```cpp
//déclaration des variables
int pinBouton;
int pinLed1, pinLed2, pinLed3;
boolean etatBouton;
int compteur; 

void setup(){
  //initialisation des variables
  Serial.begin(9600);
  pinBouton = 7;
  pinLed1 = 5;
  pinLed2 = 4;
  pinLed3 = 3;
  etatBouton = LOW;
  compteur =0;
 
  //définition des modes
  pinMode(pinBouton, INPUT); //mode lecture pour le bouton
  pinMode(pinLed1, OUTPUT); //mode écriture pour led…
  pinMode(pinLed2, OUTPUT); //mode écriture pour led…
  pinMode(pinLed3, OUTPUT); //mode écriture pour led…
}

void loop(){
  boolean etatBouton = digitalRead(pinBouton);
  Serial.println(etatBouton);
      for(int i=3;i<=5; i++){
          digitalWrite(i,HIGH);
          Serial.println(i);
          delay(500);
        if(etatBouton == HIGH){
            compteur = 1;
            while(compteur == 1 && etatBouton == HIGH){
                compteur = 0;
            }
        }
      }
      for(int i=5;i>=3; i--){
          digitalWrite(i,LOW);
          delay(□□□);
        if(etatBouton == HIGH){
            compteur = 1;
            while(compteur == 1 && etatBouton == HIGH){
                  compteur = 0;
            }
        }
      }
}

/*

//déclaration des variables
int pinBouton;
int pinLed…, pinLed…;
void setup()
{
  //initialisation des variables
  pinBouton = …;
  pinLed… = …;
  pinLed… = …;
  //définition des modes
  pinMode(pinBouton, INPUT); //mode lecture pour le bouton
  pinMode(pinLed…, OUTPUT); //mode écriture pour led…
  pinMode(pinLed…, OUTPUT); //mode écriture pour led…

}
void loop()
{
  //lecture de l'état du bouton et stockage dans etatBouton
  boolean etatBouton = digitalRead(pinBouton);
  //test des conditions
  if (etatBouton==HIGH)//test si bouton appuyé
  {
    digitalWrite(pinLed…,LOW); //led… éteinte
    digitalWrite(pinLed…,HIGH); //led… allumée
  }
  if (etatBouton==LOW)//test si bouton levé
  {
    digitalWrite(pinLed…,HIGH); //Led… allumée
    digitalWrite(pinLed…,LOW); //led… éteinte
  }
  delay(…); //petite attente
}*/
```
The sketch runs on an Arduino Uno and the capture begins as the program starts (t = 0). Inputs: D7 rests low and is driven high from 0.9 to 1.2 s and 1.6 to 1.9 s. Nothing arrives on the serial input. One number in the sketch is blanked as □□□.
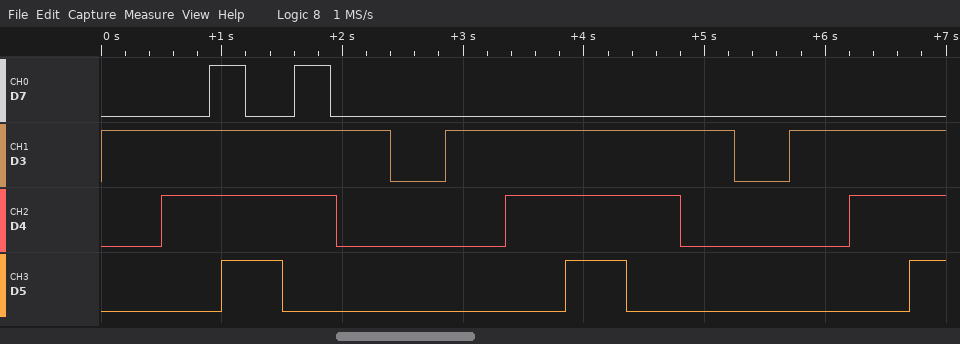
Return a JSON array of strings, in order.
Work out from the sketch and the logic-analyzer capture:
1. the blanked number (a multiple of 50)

["450"]
